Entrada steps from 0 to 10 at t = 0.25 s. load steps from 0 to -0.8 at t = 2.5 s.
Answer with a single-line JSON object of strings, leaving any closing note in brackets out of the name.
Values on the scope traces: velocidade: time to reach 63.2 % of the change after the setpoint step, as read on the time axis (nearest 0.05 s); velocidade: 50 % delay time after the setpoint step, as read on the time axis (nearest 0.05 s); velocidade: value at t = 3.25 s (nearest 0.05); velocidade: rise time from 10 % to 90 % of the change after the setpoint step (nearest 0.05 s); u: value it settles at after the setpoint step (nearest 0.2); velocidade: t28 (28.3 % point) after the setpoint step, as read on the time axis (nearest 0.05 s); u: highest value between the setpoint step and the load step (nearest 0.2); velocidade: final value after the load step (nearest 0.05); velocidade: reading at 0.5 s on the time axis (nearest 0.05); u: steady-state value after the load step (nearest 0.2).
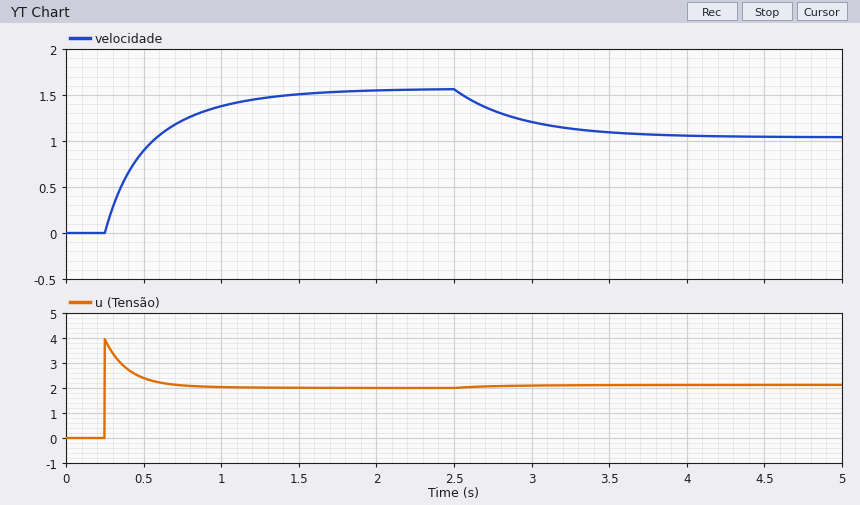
{"velocidade: time to reach 63.2 % of the change after the setpoint step, as read on the time axis": "0.55 s", "velocidade: 50 % delay time after the setpoint step, as read on the time axis": "0.45 s", "velocidade: value at t = 3.25 s": "1.15", "velocidade: rise time from 10 % to 90 % of the change after the setpoint step": "0.80 s", "u: value it settles at after the setpoint step": "2.0", "velocidade: t28 (28.3 % point) after the setpoint step, as read on the time axis": "0.35 s", "u: highest value between the setpoint step and the load step": "4.0", "velocidade: final value after the load step": "1.05", "velocidade: reading at 0.5 s on the time axis": "0.90", "u: steady-state value after the load step": "2.2"}
